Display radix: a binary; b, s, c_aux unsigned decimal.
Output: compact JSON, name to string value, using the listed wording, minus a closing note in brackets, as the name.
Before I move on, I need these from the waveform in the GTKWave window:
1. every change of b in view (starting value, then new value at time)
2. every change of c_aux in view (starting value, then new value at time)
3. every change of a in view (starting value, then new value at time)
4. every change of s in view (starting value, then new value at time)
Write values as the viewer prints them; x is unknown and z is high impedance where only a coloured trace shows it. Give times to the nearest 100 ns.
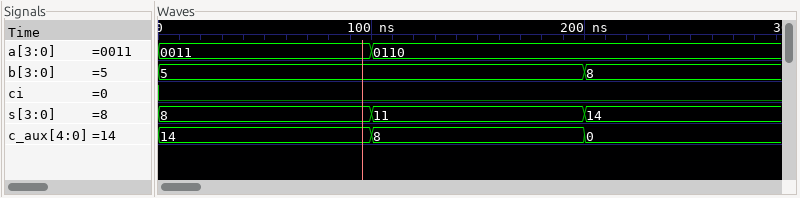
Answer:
{"every change of b in view": "5, 8 at 200 ns", "every change of c_aux in view": "14, 8 at 100 ns, 0 at 200 ns", "every change of a in view": "0011, 0110 at 100 ns", "every change of s in view": "8, 11 at 100 ns, 14 at 200 ns"}
